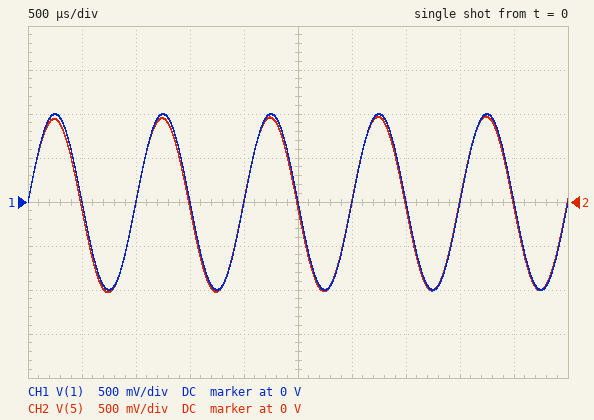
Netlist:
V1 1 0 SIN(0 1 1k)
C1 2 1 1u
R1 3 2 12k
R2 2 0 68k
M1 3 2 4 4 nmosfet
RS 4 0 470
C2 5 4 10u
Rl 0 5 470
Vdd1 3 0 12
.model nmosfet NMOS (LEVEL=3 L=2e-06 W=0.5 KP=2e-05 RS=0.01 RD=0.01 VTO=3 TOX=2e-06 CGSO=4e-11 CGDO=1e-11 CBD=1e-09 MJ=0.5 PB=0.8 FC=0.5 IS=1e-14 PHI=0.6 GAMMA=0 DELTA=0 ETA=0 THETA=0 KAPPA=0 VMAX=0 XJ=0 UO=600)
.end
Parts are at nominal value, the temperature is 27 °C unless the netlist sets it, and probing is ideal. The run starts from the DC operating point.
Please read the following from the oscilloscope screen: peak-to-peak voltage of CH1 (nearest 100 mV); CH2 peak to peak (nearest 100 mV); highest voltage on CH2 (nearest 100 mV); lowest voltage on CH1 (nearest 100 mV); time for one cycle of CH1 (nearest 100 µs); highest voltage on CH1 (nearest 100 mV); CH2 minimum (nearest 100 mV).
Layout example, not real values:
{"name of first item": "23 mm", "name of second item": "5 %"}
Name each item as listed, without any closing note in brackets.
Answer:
{"peak-to-peak voltage of CH1": "2.0 V", "CH2 peak to peak": "2.0 V", "highest voltage on CH2": "1.0 V", "lowest voltage on CH1": "-1.0 V", "time for one cycle of CH1": "1.0 ms", "highest voltage on CH1": "1.0 V", "CH2 minimum": "-1.0 V"}
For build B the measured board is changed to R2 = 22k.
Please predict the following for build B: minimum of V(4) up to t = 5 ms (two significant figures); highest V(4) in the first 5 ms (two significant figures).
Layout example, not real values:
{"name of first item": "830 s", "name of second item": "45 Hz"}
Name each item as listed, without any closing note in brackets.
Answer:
{"minimum of V(4) up to t = 5 ms": "3.7 V", "highest V(4) in the first 5 ms": "5.7 V"}
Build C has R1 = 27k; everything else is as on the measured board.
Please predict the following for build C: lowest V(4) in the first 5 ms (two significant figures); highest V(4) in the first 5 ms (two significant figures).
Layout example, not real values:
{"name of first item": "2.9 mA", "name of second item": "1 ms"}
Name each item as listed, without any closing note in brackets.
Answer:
{"lowest V(4) in the first 5 ms": "4.5 V", "highest V(4) in the first 5 ms": "6.5 V"}
